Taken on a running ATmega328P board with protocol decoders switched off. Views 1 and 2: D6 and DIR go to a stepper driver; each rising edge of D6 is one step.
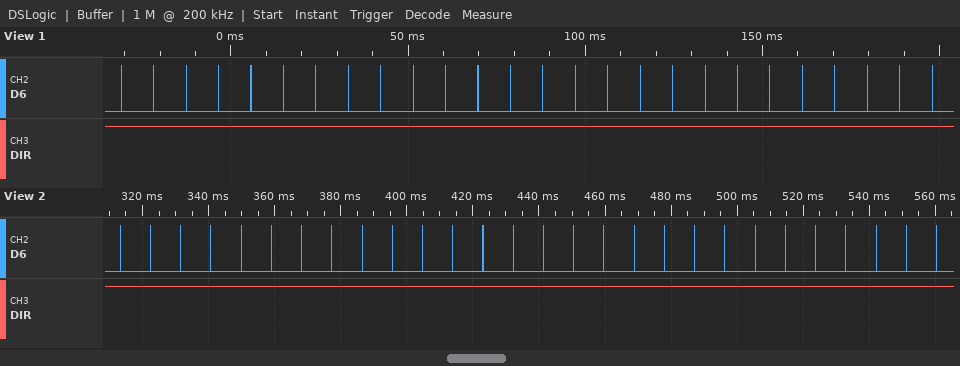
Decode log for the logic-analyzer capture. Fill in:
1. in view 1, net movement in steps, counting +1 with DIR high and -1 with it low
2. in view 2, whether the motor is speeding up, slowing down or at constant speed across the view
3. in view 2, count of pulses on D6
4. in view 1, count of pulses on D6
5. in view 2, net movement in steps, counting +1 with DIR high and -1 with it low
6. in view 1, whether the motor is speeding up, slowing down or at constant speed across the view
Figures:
+26
constant speed
28
26
+28
constant speed
